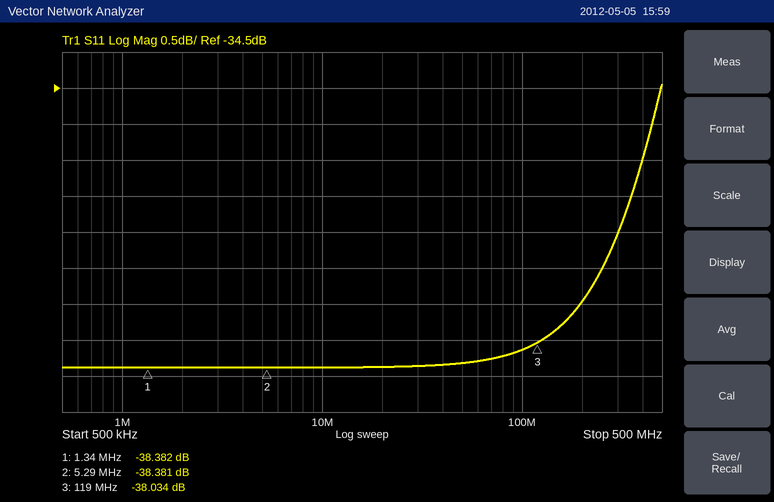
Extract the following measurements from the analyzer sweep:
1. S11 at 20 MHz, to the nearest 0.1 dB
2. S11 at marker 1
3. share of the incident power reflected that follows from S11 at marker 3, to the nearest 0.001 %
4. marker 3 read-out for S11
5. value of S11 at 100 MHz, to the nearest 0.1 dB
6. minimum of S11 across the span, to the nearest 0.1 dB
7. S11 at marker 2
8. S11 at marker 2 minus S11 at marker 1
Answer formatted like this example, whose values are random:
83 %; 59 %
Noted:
-38.4 dB; -38.382 dB; 0.016 %; -38.034 dB; -38.1 dB; -38.4 dB; -38.381 dB; 0.001 dB
